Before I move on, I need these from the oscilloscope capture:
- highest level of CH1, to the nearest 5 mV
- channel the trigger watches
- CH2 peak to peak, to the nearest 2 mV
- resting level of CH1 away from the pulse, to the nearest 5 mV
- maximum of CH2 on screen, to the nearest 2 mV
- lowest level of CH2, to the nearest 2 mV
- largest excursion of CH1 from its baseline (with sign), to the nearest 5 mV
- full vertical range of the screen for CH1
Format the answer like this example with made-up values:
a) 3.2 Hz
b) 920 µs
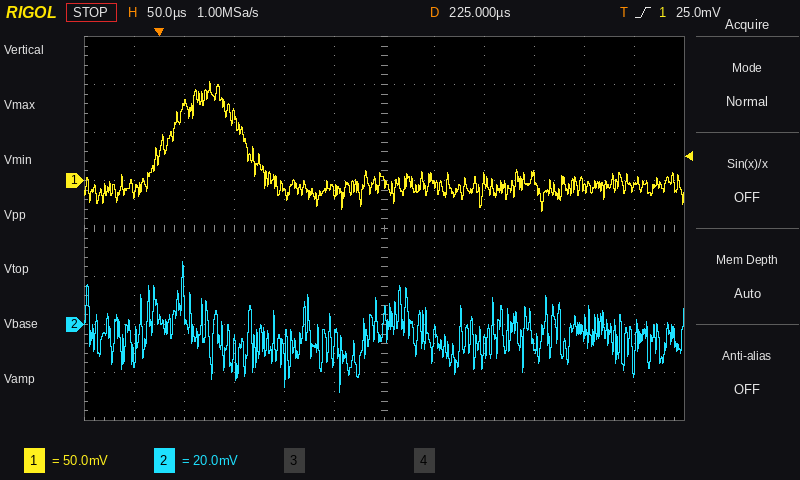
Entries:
a) 105 mV
b) CH1
c) 54 mV
d) -5 mV
e) 26 mV
f) -28 mV
g) +110 mV
h) 400 mV
